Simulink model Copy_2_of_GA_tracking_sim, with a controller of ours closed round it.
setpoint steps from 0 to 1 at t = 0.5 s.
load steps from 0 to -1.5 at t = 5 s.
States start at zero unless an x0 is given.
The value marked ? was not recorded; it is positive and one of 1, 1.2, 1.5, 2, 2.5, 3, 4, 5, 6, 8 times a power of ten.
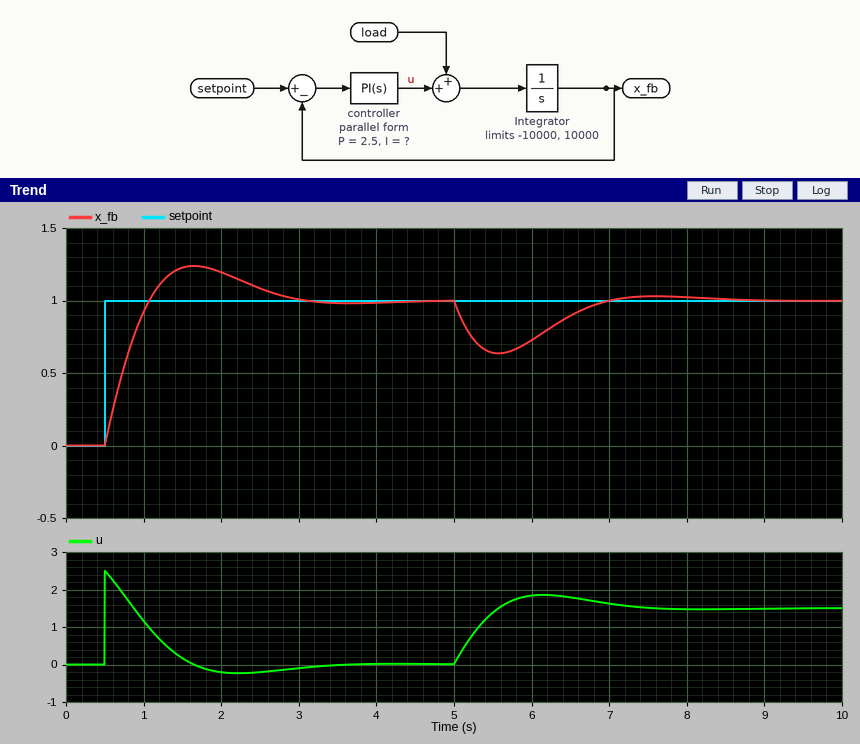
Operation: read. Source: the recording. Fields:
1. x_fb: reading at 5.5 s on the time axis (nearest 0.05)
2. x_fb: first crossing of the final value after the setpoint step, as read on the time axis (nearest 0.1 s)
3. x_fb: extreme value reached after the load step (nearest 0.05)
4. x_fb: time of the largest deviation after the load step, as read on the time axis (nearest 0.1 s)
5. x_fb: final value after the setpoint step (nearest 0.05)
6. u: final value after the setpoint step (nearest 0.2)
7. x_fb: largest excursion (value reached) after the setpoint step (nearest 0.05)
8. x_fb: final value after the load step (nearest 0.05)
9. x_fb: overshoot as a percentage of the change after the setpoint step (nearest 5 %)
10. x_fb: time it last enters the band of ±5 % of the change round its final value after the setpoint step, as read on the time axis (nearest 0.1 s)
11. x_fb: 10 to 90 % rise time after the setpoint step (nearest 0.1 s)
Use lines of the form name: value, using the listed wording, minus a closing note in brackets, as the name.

x_fb: reading at 5.5 s on the time axis: 0.65
x_fb: first crossing of the final value after the setpoint step, as read on the time axis: 1.1 s
x_fb: extreme value reached after the load step: 0.65
x_fb: time of the largest deviation after the load step, as read on the time axis: 5.6 s
x_fb: final value after the setpoint step: 1.00
u: final value after the setpoint step: 0.0
x_fb: largest excursion (value reached) after the setpoint step: 1.25
x_fb: final value after the load step: 1.00
x_fb: overshoot as a percentage of the change after the setpoint step: 25 %
x_fb: time it last enters the band of ±5 % of the change round its final value after the setpoint step, as read on the time axis: 2.7 s
x_fb: 10 to 90 % rise time after the setpoint step: 0.4 s
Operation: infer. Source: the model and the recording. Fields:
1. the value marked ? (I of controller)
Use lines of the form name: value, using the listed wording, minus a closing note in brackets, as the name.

the value marked ?: 4
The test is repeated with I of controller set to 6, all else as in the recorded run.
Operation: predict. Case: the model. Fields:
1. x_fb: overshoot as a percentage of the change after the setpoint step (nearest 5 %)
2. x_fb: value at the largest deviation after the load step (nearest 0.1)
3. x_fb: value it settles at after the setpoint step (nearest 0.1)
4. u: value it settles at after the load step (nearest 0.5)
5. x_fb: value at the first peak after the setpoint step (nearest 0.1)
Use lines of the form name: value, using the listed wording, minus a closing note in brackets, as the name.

x_fb: overshoot as a percentage of the change after the setpoint step: 30 %
x_fb: value at the largest deviation after the load step: 0.7
x_fb: value it settles at after the setpoint step: 1.0
u: value it settles at after the load step: 1.5
x_fb: value at the first peak after the setpoint step: 1.3
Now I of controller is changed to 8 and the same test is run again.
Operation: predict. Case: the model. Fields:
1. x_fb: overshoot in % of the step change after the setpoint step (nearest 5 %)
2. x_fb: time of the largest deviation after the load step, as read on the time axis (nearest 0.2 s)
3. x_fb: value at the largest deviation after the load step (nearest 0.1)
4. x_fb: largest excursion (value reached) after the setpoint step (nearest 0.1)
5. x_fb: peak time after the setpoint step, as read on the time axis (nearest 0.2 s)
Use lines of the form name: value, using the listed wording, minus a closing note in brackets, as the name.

x_fb: overshoot in % of the step change after the setpoint step: 35 %
x_fb: time of the largest deviation after the load step, as read on the time axis: 5.4 s
x_fb: value at the largest deviation after the load step: 0.7
x_fb: largest excursion (value reached) after the setpoint step: 1.3
x_fb: peak time after the setpoint step, as read on the time axis: 1.4 s
